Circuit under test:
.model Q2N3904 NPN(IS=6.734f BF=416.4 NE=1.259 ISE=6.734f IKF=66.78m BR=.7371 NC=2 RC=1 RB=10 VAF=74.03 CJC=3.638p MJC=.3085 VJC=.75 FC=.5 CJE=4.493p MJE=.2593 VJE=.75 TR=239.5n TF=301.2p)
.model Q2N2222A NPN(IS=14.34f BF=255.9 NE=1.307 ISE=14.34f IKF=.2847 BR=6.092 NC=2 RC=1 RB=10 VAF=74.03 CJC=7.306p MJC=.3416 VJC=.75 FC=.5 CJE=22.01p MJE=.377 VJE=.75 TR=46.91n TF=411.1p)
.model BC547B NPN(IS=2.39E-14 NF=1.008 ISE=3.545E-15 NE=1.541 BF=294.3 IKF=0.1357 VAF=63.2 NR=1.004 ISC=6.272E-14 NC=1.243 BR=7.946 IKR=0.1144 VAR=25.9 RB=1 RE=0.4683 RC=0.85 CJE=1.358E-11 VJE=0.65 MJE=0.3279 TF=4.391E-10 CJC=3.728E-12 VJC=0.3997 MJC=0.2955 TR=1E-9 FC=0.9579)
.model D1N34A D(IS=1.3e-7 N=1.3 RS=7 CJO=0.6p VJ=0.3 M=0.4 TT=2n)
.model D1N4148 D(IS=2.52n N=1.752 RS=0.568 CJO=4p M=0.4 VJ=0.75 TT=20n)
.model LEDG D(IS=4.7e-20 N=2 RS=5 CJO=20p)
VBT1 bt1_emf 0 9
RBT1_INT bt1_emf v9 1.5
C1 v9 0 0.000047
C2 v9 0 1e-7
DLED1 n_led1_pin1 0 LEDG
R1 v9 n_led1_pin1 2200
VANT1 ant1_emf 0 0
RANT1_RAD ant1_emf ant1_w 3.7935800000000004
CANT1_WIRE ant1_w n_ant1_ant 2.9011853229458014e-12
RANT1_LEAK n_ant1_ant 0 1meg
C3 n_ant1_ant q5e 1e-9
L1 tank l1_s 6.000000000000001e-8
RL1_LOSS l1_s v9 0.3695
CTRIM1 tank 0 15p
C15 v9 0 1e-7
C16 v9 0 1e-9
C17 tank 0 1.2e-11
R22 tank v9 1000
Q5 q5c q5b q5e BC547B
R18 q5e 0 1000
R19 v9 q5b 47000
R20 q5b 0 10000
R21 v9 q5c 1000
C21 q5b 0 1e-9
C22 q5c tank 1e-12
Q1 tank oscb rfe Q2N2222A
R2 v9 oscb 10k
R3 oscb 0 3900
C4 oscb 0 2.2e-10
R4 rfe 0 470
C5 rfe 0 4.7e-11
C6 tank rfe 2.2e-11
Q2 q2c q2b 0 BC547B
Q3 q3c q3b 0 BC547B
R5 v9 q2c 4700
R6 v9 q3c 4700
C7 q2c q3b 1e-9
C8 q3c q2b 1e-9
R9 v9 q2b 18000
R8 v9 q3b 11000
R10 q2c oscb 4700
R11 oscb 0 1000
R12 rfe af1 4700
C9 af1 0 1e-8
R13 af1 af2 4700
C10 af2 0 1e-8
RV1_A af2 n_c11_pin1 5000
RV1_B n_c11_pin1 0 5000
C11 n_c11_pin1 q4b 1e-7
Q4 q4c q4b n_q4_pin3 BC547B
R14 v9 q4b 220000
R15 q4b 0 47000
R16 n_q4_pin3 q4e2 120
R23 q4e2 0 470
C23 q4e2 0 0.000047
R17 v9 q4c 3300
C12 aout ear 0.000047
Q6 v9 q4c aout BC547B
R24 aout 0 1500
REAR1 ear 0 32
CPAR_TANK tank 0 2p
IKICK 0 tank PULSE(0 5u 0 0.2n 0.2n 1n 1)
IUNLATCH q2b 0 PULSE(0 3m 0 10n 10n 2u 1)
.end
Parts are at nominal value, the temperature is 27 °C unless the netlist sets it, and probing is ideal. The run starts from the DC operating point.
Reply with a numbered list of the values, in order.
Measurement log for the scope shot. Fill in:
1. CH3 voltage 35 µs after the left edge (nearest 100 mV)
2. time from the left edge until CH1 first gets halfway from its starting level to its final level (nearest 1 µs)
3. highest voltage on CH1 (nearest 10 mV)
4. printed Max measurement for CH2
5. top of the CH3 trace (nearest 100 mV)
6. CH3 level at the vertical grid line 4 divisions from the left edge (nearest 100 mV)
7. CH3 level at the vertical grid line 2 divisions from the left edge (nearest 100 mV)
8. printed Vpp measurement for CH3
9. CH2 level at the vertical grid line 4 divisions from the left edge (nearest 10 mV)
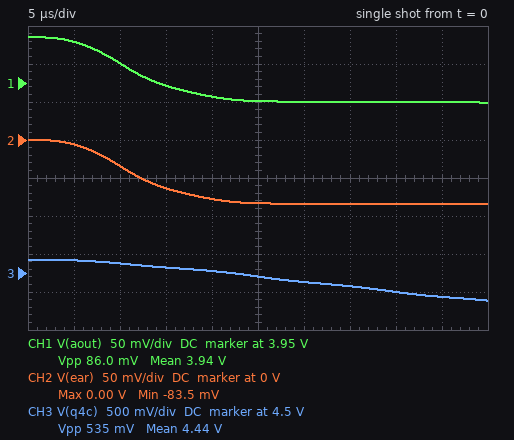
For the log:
1. 4.3 V
2. 11 µs
3. 4.01 V
4. 0.00 V
5. 4.7 V
6. 4.5 V
7. 4.6 V
8. 535 mV
9. -80 mV
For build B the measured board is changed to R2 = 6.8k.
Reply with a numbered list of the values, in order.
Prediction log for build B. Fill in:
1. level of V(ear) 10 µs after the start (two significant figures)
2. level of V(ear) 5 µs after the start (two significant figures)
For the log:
1. -38 mV
2. -7.0 mV
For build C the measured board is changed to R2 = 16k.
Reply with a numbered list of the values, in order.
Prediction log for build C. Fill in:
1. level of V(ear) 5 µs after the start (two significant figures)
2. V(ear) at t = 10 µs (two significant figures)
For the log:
1. -2.5 mV
2. -20 mV
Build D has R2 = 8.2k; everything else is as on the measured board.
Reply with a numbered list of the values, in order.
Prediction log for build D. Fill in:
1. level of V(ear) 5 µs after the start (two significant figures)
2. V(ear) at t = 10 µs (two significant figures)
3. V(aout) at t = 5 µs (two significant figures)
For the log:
1. -6.7 mV
2. -37 mV
3. 4.0 V
